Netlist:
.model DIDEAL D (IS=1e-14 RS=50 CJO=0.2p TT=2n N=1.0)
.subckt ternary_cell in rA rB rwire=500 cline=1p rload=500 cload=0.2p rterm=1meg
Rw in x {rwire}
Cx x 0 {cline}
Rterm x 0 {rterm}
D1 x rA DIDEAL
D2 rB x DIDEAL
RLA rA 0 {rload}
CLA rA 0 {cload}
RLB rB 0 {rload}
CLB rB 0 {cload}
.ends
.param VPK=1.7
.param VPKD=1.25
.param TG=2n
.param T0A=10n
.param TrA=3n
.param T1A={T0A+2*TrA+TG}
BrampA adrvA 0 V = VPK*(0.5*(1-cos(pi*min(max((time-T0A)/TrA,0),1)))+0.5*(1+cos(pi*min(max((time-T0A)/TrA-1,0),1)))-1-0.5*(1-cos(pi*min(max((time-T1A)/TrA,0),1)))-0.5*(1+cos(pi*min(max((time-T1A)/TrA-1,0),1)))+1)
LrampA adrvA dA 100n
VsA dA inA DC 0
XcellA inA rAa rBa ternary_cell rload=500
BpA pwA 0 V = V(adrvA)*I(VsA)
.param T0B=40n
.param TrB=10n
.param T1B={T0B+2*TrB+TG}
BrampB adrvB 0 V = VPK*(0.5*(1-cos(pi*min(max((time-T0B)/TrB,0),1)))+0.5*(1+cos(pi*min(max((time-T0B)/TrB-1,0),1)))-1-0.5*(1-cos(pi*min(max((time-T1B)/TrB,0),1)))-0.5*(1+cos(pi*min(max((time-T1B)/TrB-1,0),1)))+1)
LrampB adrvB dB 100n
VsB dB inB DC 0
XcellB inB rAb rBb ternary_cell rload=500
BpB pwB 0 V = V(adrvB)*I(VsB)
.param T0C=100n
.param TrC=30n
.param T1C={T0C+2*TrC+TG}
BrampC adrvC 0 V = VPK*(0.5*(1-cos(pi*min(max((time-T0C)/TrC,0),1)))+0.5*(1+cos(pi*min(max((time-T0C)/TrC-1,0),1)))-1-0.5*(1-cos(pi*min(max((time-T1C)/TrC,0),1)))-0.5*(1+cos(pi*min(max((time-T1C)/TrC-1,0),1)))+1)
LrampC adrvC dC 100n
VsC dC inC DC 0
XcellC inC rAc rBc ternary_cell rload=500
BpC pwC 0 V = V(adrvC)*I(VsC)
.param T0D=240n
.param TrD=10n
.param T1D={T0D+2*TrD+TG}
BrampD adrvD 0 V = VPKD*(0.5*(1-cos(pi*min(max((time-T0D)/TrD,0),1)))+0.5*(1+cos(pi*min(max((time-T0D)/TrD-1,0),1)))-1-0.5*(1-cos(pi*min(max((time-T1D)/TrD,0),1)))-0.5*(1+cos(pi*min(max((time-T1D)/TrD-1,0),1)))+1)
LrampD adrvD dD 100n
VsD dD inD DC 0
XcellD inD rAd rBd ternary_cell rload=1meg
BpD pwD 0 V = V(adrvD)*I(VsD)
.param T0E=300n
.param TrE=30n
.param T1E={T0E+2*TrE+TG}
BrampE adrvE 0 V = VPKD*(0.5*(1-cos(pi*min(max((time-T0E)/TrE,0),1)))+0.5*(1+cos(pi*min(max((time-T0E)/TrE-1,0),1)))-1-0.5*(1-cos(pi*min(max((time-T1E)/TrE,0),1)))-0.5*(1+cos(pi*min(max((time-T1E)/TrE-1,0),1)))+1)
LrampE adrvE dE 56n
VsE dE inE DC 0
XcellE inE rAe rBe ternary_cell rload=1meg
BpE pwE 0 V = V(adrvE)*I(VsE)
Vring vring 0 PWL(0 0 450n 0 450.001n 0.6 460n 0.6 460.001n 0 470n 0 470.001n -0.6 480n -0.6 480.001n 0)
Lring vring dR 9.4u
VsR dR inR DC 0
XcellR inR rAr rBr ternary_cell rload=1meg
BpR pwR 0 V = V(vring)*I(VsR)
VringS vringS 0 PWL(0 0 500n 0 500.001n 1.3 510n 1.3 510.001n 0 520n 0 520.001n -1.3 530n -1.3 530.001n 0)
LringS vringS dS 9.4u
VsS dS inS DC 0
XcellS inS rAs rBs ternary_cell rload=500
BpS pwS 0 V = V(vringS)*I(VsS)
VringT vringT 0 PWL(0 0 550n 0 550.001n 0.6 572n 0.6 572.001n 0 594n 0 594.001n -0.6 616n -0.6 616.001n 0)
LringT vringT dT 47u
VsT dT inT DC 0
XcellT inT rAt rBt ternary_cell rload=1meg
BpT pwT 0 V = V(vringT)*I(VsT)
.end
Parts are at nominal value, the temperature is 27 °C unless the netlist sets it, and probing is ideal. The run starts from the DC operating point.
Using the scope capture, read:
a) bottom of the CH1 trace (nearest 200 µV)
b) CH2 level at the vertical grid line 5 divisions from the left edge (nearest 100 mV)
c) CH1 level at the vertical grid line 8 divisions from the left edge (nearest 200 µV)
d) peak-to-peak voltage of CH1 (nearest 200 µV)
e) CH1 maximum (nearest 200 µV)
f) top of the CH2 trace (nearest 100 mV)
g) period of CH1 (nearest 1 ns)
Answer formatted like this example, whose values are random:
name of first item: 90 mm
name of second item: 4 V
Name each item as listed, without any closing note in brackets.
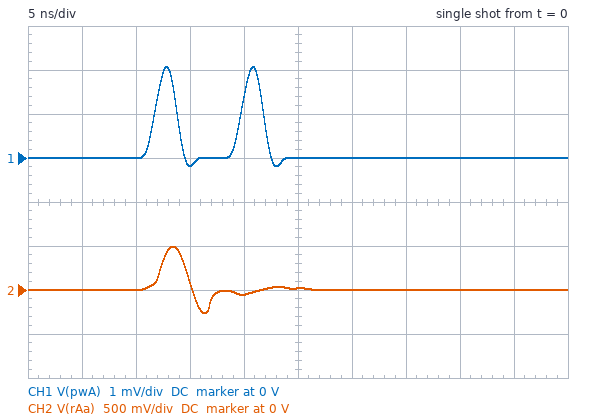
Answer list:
bottom of the CH1 trace: -200 µV
CH2 level at the vertical grid line 5 divisions from the left edge: 0 V
CH1 level at the vertical grid line 8 divisions from the left edge: 0 V
peak-to-peak voltage of CH1: 2.2 mV
CH1 maximum: 2.0 mV
top of the CH2 trace: 500 mV
period of CH1: 8 ns
